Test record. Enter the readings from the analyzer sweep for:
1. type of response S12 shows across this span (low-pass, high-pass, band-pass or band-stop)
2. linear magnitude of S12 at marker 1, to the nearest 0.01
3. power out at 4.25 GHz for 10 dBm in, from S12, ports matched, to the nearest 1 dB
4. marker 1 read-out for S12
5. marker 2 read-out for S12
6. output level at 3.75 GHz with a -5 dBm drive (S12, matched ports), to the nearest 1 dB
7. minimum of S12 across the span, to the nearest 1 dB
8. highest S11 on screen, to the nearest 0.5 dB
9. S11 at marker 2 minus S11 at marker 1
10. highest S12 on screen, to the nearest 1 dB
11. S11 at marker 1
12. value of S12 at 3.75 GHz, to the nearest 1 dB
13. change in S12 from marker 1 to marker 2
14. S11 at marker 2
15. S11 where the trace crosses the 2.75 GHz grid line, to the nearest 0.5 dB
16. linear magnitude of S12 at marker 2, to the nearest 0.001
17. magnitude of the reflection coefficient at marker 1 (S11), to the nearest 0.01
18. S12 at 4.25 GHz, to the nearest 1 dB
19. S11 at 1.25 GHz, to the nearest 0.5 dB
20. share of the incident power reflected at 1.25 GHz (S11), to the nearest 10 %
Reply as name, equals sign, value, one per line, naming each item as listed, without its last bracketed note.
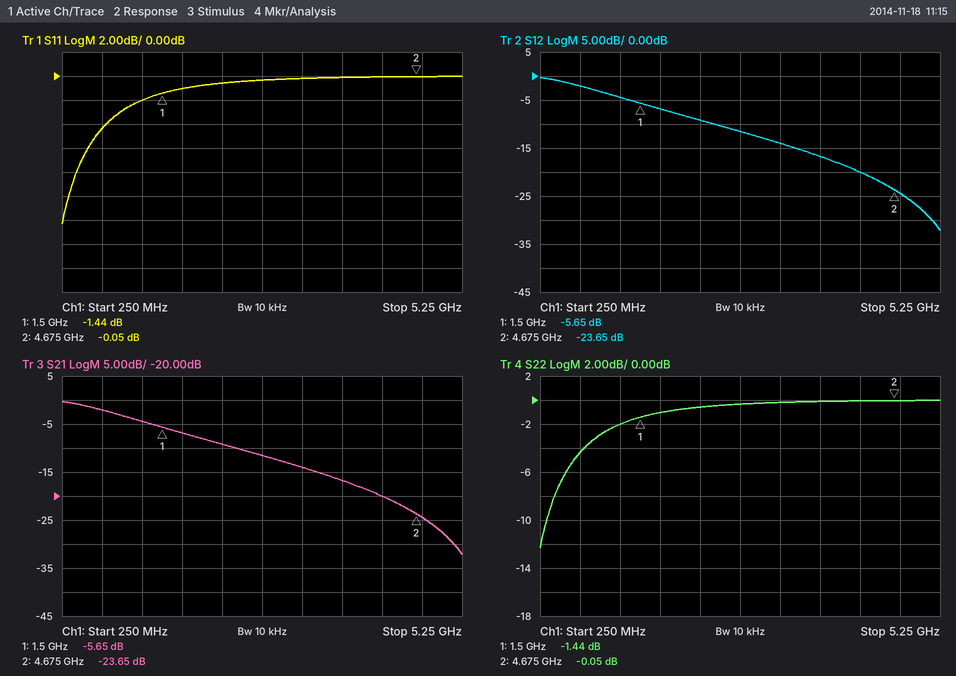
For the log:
type of response S12 shows across this span = low-pass
linear magnitude of S12 at marker 1, to the nearest 0.01 = 0.52
power out at 4.25 GHz for 10 dBm in, from S12, ports matched, to the nearest 1 dB = -10 dBm
marker 1 read-out for S12 = -5.65 dB
marker 2 read-out for S12 = -23.65 dB
output level at 3.75 GHz with a -5 dBm drive (S12, matched ports), to the nearest 1 dB = -22 dBm
minimum of S12 across the span, to the nearest 1 dB = -32 dB
highest S11 on screen, to the nearest 0.5 dB = 0.0 dB
S11 at marker 2 minus S11 at marker 1 = 1.39 dB
highest S12 on screen, to the nearest 1 dB = 0 dB
S11 at marker 1 = -1.44 dB
value of S12 at 3.75 GHz, to the nearest 1 dB = -17 dB
change in S12 from marker 1 to marker 2 = -18.00 dB
S11 at marker 2 = -0.05 dB
S11 where the trace crosses the 2.75 GHz grid line, to the nearest 0.5 dB = -0.5 dB
linear magnitude of S12 at marker 2, to the nearest 0.001 = 0.066
magnitude of the reflection coefficient at marker 1 (S11), to the nearest 0.01 = 0.85
S12 at 4.25 GHz, to the nearest 1 dB = -20 dB
S11 at 1.25 GHz, to the nearest 0.5 dB = -2.0 dB
share of the incident power reflected at 1.25 GHz (S11), to the nearest 10 % = 60 %
